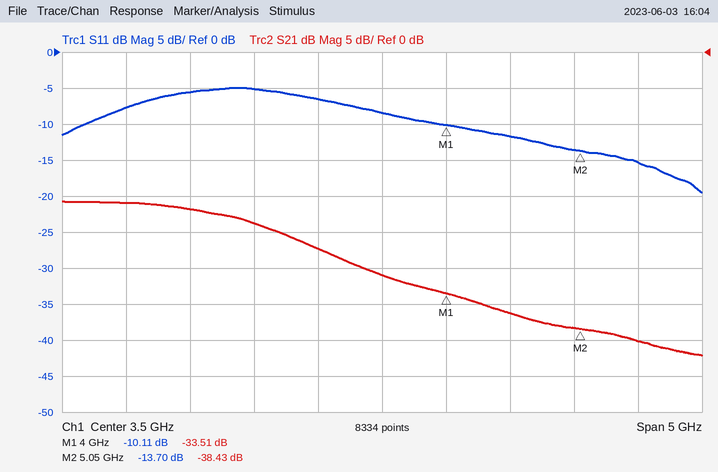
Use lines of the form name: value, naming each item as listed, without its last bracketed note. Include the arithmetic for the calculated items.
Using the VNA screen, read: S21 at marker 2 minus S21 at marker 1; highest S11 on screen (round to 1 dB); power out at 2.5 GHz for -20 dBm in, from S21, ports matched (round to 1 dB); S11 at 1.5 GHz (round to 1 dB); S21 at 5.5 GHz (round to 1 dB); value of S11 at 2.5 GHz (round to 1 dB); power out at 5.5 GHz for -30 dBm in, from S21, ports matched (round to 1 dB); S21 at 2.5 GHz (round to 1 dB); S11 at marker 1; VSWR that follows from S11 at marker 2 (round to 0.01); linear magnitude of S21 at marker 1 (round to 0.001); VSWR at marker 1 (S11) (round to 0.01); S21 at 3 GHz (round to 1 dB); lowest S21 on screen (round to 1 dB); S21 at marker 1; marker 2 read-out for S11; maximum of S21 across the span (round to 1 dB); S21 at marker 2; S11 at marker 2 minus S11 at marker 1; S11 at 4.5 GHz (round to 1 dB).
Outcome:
S21 at marker 2 minus S21 at marker 1: -38.43 − (-33.51) = -4.92 dB
highest S11 on screen: -5 dB
power out at 2.5 GHz for -20 dBm in, from S21, ports matched: -20 dBm + (-24 dB) = -44 dBm
S11 at 1.5 GHz: -8 dB
S21 at 5.5 GHz: -40 dB
value of S11 at 2.5 GHz: -5 dB
power out at 5.5 GHz for -30 dBm in, from S21, ports matched: -30 dBm + (-40 dB) = -70 dBm
S21 at 2.5 GHz: -24 dB
S11 at marker 1: -10.11 dB
VSWR that follows from S11 at marker 2: (1 + 0.2065)/(1 − 0.2065) ≈ 1.52
linear magnitude of S21 at marker 1: 10^(-33.51/20) ≈ 0.021
VSWR at marker 1 (S11): (1 + 0.3122)/(1 − 0.3122) ≈ 1.91
S21 at 3 GHz: -27 dB
lowest S21 on screen: -42 dB
S21 at marker 1: -33.51 dB
marker 2 read-out for S11: -13.70 dB
maximum of S21 across the span: -21 dB
S21 at marker 2: -38.43 dB
S11 at marker 2 minus S11 at marker 1: -13.7 − (-10.11) = -3.59 dB
S11 at 4.5 GHz: -12 dB
